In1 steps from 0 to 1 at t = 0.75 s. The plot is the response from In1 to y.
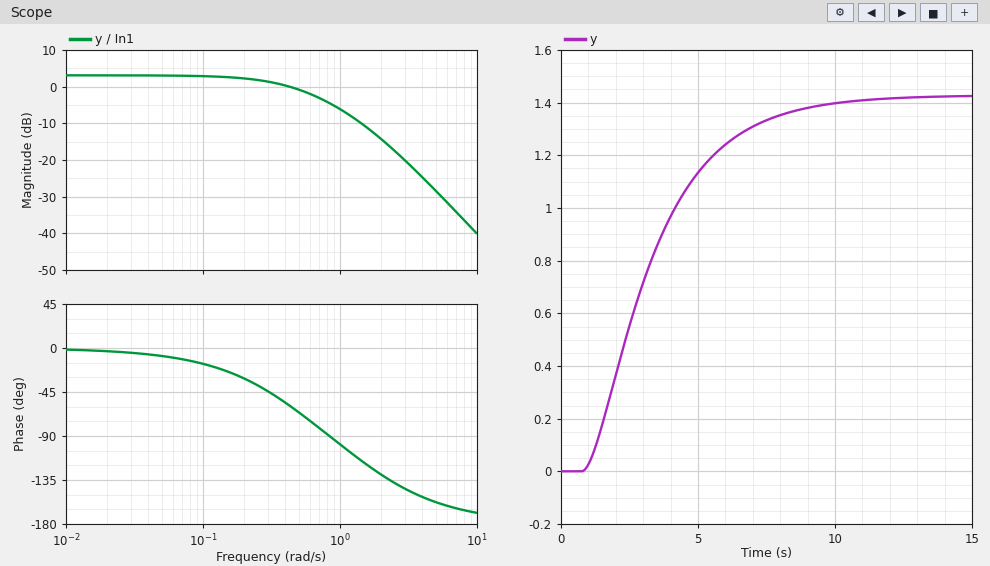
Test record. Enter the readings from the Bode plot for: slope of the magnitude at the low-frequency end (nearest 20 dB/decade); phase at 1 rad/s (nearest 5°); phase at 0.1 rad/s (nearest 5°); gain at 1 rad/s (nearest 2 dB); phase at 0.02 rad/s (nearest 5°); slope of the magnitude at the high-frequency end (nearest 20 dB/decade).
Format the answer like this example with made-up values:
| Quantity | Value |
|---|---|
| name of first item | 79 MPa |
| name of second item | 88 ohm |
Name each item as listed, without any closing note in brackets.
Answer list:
| Quantity | Value |
|---|---|
| slope of the magnitude at the low-frequency end | 0 dB/decade |
| phase at 1 rad/s | -100° |
| phase at 0.1 rad/s | -15° |
| gain at 1 rad/s | -6 dB |
| phase at 0.02 rad/s | -5° |
| slope of the magnitude at the high-frequency end | -40 dB/decade |
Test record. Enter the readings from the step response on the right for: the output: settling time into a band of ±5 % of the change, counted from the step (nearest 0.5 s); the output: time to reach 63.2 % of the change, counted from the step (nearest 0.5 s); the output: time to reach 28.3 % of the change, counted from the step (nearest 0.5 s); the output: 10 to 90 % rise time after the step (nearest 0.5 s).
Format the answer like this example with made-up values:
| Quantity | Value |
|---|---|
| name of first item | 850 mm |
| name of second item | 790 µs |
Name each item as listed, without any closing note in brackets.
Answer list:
| Quantity | Value |
|---|---|
| the output: settling time into a band of ±5 % of the change, counted from the step | 7.5 s |
| the output: time to reach 63.2 % of the change, counted from the step | 3.0 s |
| the output: time to reach 28.3 % of the change, counted from the step | 1.5 s |
| the output: 10 to 90 % rise time after the step | 5.0 s |
